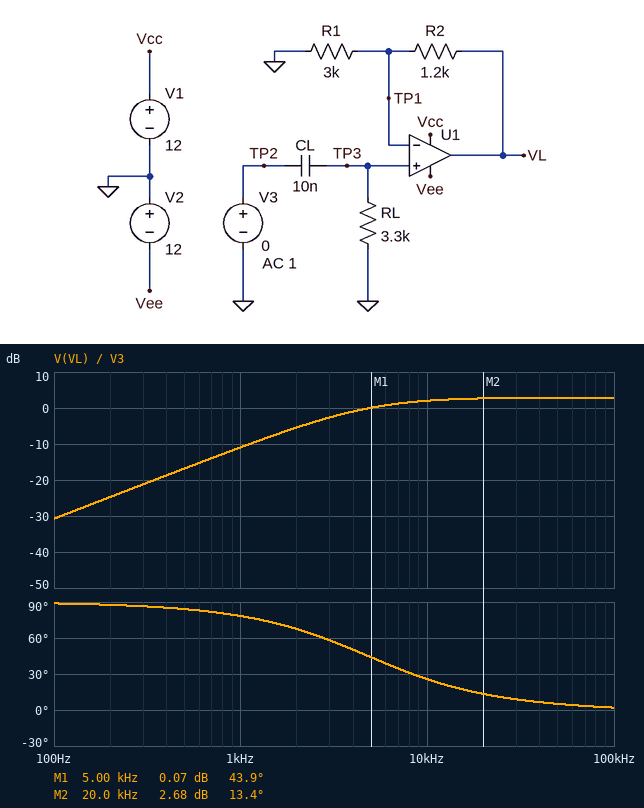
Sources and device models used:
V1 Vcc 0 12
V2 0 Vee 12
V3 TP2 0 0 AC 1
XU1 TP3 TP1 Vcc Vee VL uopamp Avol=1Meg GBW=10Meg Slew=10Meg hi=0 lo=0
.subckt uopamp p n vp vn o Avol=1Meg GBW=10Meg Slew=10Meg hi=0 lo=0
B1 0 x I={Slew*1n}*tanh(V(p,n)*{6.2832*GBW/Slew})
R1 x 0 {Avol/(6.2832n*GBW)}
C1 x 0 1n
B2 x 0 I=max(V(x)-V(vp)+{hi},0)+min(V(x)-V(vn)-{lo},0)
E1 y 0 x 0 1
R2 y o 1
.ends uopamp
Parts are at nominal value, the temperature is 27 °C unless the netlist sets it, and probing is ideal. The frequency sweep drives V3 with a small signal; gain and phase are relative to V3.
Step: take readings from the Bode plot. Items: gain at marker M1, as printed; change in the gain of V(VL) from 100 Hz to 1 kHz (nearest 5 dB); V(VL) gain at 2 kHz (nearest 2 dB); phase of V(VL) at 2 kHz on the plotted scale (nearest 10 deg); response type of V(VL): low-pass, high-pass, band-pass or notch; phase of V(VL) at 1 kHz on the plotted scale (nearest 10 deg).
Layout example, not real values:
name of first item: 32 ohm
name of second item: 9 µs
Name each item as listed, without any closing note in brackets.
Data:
gain at marker M1, as printed: 0.07 dB
change in the gain of V(VL) from 100 Hz to 1 kHz: 20 dB
V(VL) gain at 2 kHz: -6 dB
phase of V(VL) at 2 kHz on the plotted scale: 70 deg
response type of V(VL): low-pass, high-pass, band-pass or notch: high-pass
phase of V(VL) at 1 kHz on the plotted scale: 80 deg
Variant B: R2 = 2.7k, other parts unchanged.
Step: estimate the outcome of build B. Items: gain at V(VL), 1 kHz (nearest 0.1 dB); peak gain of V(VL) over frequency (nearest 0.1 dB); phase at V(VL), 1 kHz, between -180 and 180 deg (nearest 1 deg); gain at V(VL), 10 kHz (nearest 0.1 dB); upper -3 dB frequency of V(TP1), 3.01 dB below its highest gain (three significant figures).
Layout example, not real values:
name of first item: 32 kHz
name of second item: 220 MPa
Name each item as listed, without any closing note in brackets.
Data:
gain at V(VL), 1 kHz: -8.3 dB
peak gain of V(VL) over frequency: 5.6 dB
phase at V(VL), 1 kHz, between -180 and 180 deg: 78 deg
gain at V(VL), 10 kHz: 4.7 dB
upper -3 dB frequency of V(TP1), 3.01 dB below its highest gain: 5.27 MHz
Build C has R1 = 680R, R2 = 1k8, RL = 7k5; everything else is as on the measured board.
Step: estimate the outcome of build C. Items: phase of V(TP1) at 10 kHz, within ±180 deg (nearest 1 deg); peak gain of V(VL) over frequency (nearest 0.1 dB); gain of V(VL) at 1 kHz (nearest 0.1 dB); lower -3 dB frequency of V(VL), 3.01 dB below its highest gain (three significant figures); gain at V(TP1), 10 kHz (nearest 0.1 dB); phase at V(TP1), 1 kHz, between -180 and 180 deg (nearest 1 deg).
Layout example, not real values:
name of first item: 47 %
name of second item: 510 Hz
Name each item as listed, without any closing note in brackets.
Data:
phase of V(TP1) at 10 kHz, within ±180 deg: 12 deg
peak gain of V(VL) over frequency: 11.2 dB
gain of V(VL) at 1 kHz: 3.8 dB
lower -3 dB frequency of V(VL), 3.01 dB below its highest gain: 2.12 kHz
gain at V(TP1), 10 kHz: -0.2 dB
phase at V(TP1), 1 kHz, between -180 and 180 deg: 65 deg
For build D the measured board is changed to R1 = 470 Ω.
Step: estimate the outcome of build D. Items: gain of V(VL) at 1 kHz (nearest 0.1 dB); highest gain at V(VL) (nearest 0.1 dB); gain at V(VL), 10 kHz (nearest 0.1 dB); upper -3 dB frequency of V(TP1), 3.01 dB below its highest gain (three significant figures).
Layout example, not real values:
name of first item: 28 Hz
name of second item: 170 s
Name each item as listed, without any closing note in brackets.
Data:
gain of V(VL) at 1 kHz: -2.8 dB
highest gain at V(VL): 11.0 dB
gain at V(VL), 10 kHz: 10.1 dB
upper -3 dB frequency of V(TP1), 3.01 dB below its highest gain: 2.82 MHz
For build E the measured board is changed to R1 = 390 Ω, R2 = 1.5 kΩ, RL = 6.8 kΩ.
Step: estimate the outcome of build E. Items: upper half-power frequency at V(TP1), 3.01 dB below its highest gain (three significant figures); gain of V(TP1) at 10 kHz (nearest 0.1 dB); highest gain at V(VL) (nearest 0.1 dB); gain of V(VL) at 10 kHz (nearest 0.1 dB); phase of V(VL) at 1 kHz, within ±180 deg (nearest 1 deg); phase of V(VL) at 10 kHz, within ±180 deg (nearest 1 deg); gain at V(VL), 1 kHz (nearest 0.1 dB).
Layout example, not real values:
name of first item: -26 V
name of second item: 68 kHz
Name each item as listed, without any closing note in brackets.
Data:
upper half-power frequency at V(TP1), 3.01 dB below its highest gain: 2.07 MHz
gain of V(TP1) at 10 kHz: -0.2 dB
highest gain at V(VL): 13.7 dB
gain of V(VL) at 10 kHz: 13.5 dB
phase of V(VL) at 1 kHz, within ±180 deg: 67 deg
phase of V(VL) at 10 kHz, within ±180 deg: 13 deg
gain at V(VL), 1 kHz: 5.6 dB
